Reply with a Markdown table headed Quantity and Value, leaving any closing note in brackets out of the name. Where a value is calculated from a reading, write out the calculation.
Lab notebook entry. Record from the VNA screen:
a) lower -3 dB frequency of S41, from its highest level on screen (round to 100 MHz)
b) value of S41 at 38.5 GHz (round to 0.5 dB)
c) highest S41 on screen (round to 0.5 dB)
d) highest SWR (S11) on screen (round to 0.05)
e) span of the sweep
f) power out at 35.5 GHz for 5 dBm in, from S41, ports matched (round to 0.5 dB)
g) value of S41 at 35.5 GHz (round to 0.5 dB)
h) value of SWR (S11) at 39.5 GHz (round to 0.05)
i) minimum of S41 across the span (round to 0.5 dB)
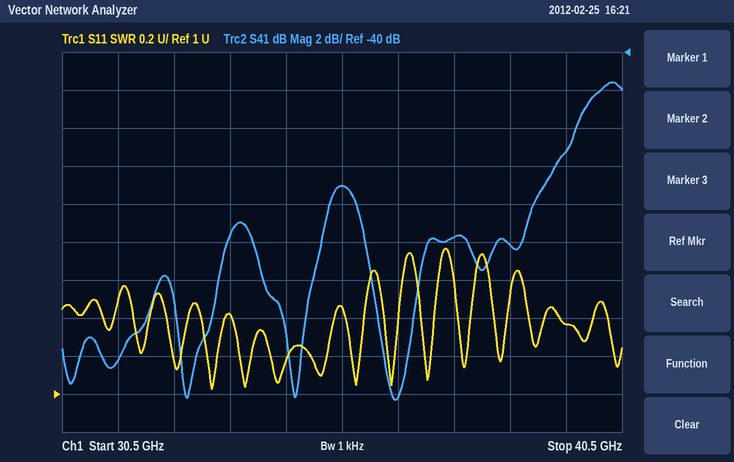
| Quantity | Value |
|---|---|
| lower -3 dB frequency of S41, from its highest level on screen | 39.6 GHz |
| value of S41 at 38.5 GHz | -50.0 dB |
| highest S41 on screen | -41.5 dB |
| highest SWR (S11) on screen | 1.75 |
| span of the sweep | 10 GHz |
| power out at 35.5 GHz for 5 dBm in, from S41, ports matched | 5 dBm + (-47.0 dB) = -42.0 dBm |
| value of S41 at 35.5 GHz | -47.0 dB |
| value of SWR (S11) at 39.5 GHz | 1.35 |
| minimum of S41 across the span | -58.5 dB |
